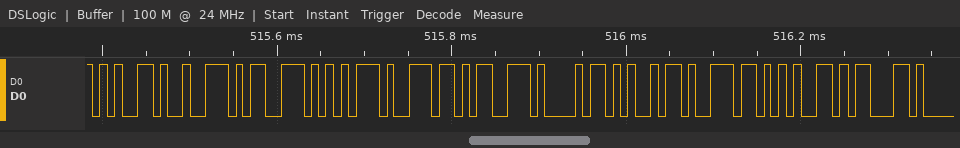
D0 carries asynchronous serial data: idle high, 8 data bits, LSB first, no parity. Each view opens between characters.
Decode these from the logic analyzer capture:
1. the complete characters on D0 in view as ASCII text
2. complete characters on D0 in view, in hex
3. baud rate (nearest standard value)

"ersunshinec"
65, 72, 73, 75, 6E, 73, 68, 69, 6E, 65, 63
115200 baud
